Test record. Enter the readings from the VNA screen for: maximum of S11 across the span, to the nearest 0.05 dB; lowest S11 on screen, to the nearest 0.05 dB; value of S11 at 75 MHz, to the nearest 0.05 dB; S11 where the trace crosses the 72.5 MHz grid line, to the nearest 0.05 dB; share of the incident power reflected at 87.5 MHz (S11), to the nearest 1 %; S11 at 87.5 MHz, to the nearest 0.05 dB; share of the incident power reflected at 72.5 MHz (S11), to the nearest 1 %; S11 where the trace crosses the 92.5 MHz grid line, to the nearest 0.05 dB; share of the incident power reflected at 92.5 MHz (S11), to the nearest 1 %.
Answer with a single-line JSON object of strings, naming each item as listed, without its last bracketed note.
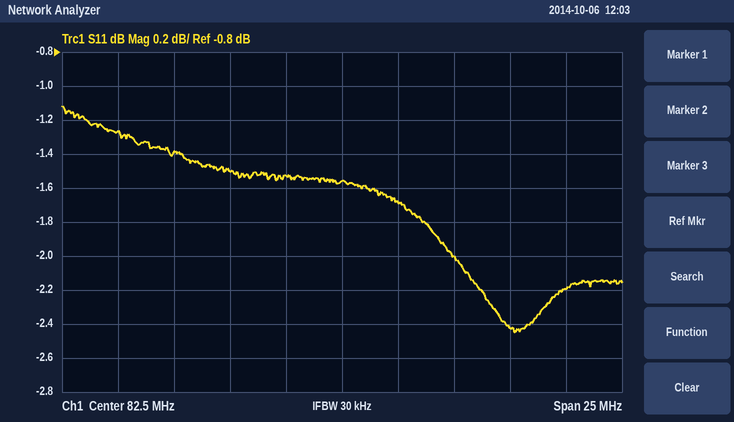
{"maximum of S11 across the span, to the nearest 0.05 dB": "-1.10 dB", "lowest S11 on screen, to the nearest 0.05 dB": "-2.45 dB", "value of S11 at 75 MHz, to the nearest 0.05 dB": "-1.40 dB", "S11 where the trace crosses the 72.5 MHz grid line, to the nearest 0.05 dB": "-1.25 dB", "share of the incident power reflected at 87.5 MHz (S11), to the nearest 1 %": "63 %", "S11 at 87.5 MHz, to the nearest 0.05 dB": "-2.00 dB", "share of the incident power reflected at 72.5 MHz (S11), to the nearest 1 %": "75 %", "S11 where the trace crosses the 92.5 MHz grid line, to the nearest 0.05 dB": "-2.20 dB", "share of the incident power reflected at 92.5 MHz (S11), to the nearest 1 %": "60 %"}
